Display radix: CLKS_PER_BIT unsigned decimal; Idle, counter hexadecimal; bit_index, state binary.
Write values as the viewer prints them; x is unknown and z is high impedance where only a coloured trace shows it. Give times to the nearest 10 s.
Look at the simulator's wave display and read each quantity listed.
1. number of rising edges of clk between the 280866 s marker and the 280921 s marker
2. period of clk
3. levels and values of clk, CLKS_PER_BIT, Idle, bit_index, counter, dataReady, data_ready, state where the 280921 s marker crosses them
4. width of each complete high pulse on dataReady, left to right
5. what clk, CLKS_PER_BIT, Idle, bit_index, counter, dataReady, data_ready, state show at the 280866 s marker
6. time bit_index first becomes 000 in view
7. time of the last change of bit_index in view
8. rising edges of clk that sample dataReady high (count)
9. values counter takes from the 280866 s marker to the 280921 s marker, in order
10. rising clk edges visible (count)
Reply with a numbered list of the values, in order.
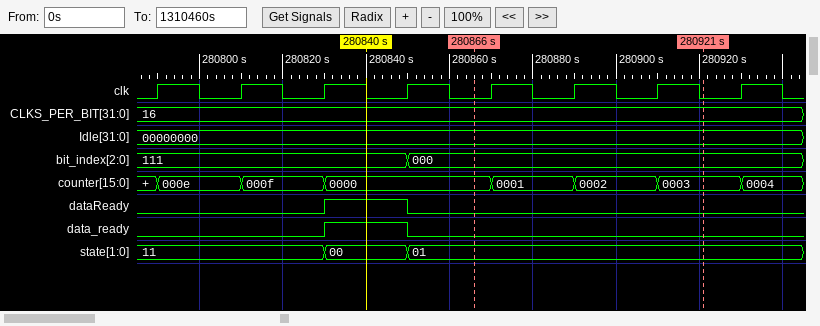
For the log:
1. 3
2. 20 s
3. clk=0, CLKS_PER_BIT=16, Idle=00000000, bit_index=000, counter=0003, dataReady=0, data_ready=0, state=01
4. 20 s
5. clk=0, CLKS_PER_BIT=16, Idle=00000000, bit_index=000, counter=0000, dataReady=0, data_ready=0, state=01
6. 280850 s
7. 280850 s
8. 1
9. 0000, 0001, 0002, 0003
10. 8
